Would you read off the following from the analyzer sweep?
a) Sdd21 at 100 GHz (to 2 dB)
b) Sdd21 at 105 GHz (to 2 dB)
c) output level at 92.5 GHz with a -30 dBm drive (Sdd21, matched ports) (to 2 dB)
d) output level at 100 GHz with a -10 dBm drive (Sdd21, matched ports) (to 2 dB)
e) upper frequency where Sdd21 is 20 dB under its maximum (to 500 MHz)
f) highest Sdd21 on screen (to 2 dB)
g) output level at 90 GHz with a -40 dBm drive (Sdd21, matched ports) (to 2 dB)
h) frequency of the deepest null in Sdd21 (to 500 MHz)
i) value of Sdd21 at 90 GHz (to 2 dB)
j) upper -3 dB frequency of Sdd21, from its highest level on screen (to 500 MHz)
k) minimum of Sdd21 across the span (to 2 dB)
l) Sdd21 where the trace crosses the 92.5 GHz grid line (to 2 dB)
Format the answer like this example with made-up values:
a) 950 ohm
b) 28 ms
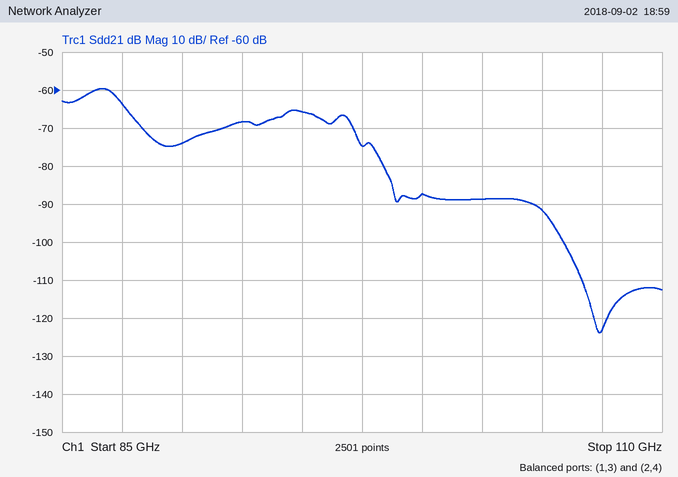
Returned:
a) -88 dB
b) -92 dB
c) -98 dBm
d) -98 dBm
e) 98.5 GHz
f) -60 dB
g) -114 dBm
h) 107.5 GHz
i) -74 dB
j) 87.5 GHz
k) -124 dB
l) -68 dB
